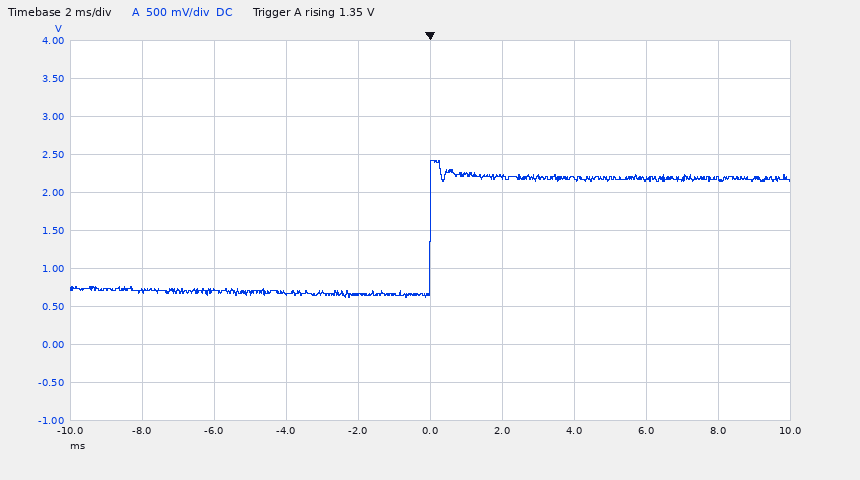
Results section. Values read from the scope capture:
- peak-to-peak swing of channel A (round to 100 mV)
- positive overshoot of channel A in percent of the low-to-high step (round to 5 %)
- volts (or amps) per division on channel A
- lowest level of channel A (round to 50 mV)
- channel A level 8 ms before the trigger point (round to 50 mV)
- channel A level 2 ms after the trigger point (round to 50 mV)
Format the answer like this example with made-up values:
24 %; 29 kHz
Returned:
1.80 V; 15 %; 500 mV; 600 mV; 700 mV; 2.20 V
